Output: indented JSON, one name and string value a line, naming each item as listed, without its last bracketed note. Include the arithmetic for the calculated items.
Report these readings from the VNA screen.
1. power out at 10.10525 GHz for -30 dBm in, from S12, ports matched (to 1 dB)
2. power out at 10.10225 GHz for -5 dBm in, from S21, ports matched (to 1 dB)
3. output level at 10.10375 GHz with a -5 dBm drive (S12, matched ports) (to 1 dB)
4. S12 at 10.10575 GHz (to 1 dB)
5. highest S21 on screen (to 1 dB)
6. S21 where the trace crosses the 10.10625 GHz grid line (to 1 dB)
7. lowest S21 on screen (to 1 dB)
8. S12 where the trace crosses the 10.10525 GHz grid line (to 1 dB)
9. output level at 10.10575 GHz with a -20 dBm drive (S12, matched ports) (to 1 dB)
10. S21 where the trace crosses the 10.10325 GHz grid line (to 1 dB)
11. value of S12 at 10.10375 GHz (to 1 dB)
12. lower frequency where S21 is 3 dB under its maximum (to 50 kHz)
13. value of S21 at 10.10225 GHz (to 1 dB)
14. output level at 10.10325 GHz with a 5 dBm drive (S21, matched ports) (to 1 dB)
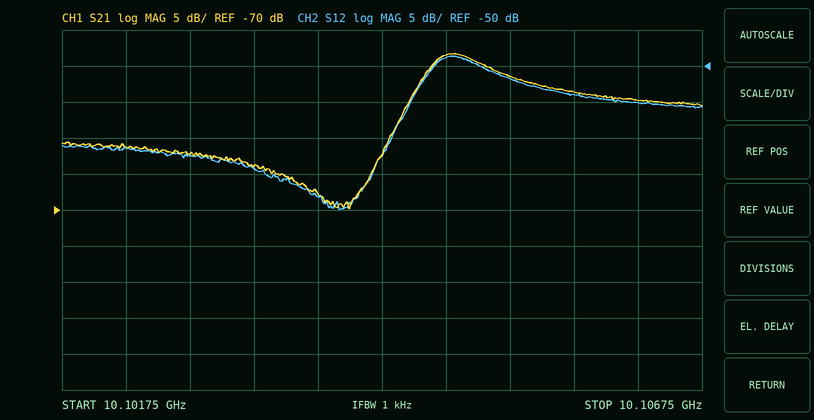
{
  "power out at 10.10525 GHz for -30 dBm in, from S12, ports matched": "-30 dBm + (-52 dB) = -82 dBm",
  "power out at 10.10225 GHz for -5 dBm in, from S21, ports matched": "-5 dBm + (-61 dB) = -66 dBm",
  "output level at 10.10375 GHz with a -5 dBm drive (S12, matched ports)": "-5 dBm + (-68 dB) = -73 dBm",
  "S12 at 10.10575 GHz": "-54 dB",
  "highest S21 on screen": "-48 dB",
  "S21 where the trace crosses the 10.10625 GHz grid line": "-55 dB",
  "lowest S21 on screen": "-70 dB",
  "S12 where the trace crosses the 10.10525 GHz grid line": "-52 dB",
  "output level at 10.10575 GHz with a -20 dBm drive (S12, matched ports)": "-20 dBm + (-54 dB) = -74 dBm",
  "S21 where the trace crosses the 10.10325 GHz grid line": "-64 dB",
  "value of S12 at 10.10375 GHz": "-68 dB",
  "lower frequency where S21 is 3 dB under its maximum": "10.10460 GHz",
  "value of S21 at 10.10225 GHz": "-61 dB",
  "output level at 10.10325 GHz with a 5 dBm drive (S21, matched ports)": "5 dBm + (-64 dB) = -59 dBm"
}
